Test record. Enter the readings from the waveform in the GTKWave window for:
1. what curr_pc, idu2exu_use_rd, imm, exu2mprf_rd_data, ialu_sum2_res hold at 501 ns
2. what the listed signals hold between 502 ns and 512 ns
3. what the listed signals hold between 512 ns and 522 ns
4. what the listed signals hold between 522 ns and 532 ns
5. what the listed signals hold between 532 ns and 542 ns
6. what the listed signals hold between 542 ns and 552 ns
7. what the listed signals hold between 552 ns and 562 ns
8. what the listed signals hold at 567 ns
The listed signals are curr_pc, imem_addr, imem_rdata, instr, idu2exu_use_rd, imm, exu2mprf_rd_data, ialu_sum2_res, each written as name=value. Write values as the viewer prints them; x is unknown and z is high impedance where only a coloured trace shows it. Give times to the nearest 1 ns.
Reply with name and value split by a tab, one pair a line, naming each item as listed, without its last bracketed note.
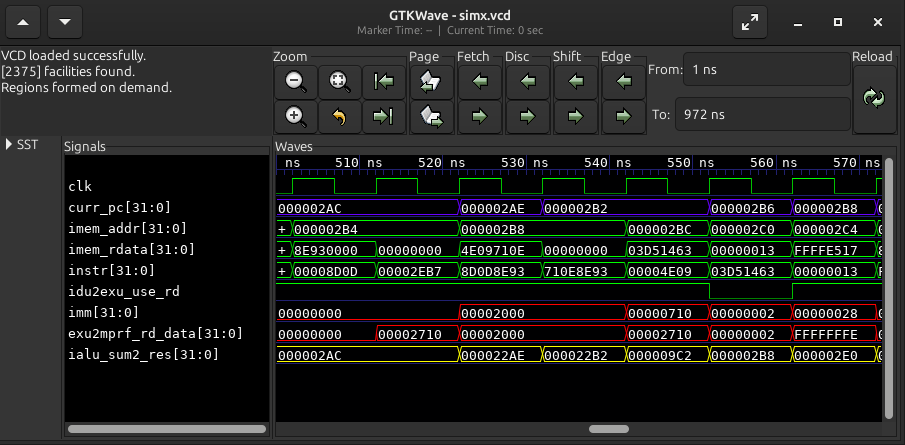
what curr_pc, idu2exu_use_rd, imm, exu2mprf_rd_data, ialu_sum2_res hold at 501 ns	curr_pc=000002AC, idu2exu_use_rd=1, imm=00000000, exu2mprf_rd_data=00000000, ialu_sum2_res=000002AC
what the listed signals hold between 502 ns and 512 ns	curr_pc=000002AC, imem_addr=000002B4, imem_rdata=8E930000, instr=00008D0D, idu2exu_use_rd=1, imm=00000000, exu2mprf_rd_data=00000000, ialu_sum2_res=000002AC
what the listed signals hold between 512 ns and 522 ns	curr_pc=000002AC, imem_addr=000002B4, imem_rdata=00000000, instr=00002EB7, idu2exu_use_rd=1, imm=00000000, exu2mprf_rd_data=00002710, ialu_sum2_res=000002AC
what the listed signals hold between 522 ns and 532 ns	curr_pc=000002AE, imem_addr=000002B8, imem_rdata=4E09710E, instr=8D0D8E93, idu2exu_use_rd=1, imm=00002000, exu2mprf_rd_data=00002000, ialu_sum2_res=000022AE
what the listed signals hold between 532 ns and 542 ns	curr_pc=000002B2, imem_addr=000002B8, imem_rdata=00000000, instr=710E8E93, idu2exu_use_rd=1, imm=00002000, exu2mprf_rd_data=00002000, ialu_sum2_res=000022B2
what the listed signals hold between 542 ns and 552 ns	curr_pc=000002B2, imem_addr=000002BC, imem_rdata=03D51463, instr=00004E09, idu2exu_use_rd=1, imm=00000710, exu2mprf_rd_data=00002710, ialu_sum2_res=000009C2
what the listed signals hold between 552 ns and 562 ns	curr_pc=000002B6, imem_addr=000002C0, imem_rdata=00000013, instr=03D51463, idu2exu_use_rd=0, imm=00000002, exu2mprf_rd_data=00000002, ialu_sum2_res=000002B8
what the listed signals hold at 567 ns	curr_pc=000002B8, imem_addr=000002C4, imem_rdata=FFFFE517, instr=00000013, idu2exu_use_rd=1, imm=00000028, exu2mprf_rd_data=FFFFFFFE, ialu_sum2_res=000002E0
